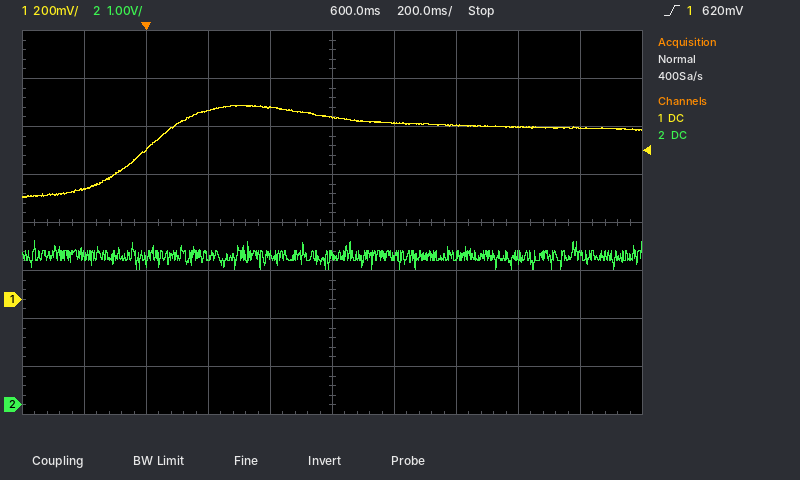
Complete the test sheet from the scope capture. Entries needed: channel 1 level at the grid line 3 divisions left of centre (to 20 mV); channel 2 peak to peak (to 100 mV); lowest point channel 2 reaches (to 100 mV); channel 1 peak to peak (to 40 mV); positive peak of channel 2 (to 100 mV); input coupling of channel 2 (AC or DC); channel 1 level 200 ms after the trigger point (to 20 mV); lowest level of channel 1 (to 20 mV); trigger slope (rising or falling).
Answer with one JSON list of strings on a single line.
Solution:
["620 mV", "600 mV", "2.8 V", "400 mV", "3.4 V", "DC", "780 mV", "420 mV", "rising"]
